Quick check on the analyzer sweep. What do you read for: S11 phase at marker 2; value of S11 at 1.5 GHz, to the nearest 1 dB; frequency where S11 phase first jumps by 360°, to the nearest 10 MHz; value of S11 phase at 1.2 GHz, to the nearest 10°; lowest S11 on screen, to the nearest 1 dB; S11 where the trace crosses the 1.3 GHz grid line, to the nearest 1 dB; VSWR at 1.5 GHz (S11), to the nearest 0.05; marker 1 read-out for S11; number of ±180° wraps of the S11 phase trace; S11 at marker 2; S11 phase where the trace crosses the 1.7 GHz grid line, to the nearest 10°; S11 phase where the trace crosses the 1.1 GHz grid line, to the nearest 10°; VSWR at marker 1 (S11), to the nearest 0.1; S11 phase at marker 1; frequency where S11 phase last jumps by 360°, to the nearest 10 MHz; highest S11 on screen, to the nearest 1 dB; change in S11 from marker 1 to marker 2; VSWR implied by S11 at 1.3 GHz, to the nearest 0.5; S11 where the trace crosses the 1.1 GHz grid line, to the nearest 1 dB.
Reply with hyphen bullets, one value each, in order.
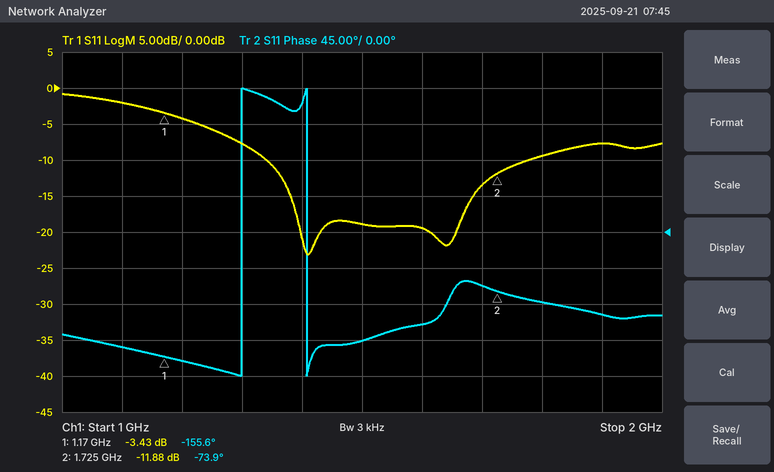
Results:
- -73.9°
- -19 dB
- 1.30 GHz
- -160°
- -23 dB
- -8 dB
- 1.25
- -3.43 dB
- 2
- -11.88 dB
- -70°
- -140°
- 5.1
- -155.6°
- 1.41 GHz
- -1 dB
- -8.45 dB
- 2.5
- -2 dB
